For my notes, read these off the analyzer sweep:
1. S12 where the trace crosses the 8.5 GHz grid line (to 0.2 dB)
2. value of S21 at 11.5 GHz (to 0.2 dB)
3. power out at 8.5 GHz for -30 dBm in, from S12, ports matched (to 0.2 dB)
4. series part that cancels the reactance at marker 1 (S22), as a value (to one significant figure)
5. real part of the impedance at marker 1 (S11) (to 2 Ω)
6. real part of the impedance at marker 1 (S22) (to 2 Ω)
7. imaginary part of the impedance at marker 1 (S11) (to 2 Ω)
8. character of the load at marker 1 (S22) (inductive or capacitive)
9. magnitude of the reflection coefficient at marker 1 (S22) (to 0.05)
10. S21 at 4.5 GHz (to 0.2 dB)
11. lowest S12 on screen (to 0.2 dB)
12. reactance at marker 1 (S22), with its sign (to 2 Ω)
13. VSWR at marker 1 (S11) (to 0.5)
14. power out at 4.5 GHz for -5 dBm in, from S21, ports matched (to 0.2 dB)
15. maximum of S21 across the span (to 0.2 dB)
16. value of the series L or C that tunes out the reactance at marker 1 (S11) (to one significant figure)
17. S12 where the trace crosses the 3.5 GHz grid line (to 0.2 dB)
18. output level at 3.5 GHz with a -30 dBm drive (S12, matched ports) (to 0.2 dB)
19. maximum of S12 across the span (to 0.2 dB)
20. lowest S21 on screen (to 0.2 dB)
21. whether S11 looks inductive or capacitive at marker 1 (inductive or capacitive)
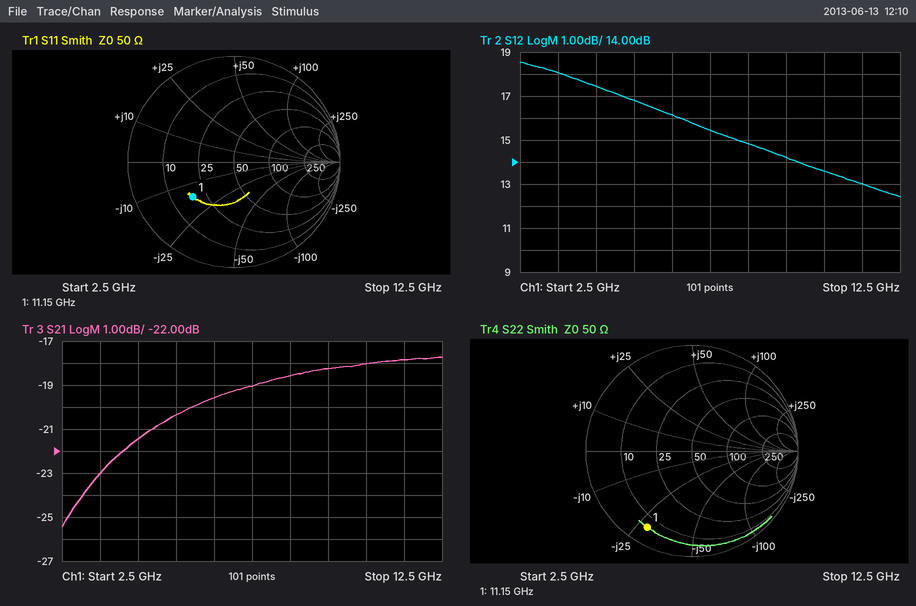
14.8 dB
-17.8 dB
-15.2 dBm
400 pH
18 Ω
6 Ω
-16 Ω
capacitive
0.85
-21.4 dB
12.4 dB
-28 Ω
3.0
-26.4 dBm
-17.8 dB
200 pH
18.0 dB
-12.0 dBm
18.6 dB
-25.4 dB
capacitive
